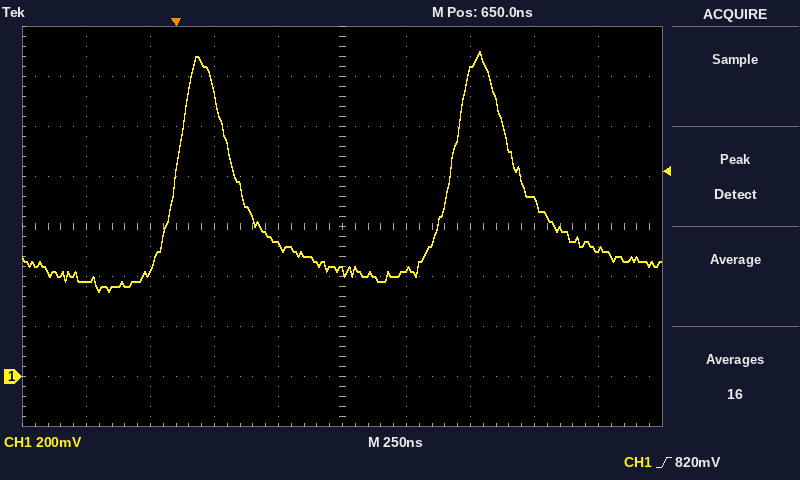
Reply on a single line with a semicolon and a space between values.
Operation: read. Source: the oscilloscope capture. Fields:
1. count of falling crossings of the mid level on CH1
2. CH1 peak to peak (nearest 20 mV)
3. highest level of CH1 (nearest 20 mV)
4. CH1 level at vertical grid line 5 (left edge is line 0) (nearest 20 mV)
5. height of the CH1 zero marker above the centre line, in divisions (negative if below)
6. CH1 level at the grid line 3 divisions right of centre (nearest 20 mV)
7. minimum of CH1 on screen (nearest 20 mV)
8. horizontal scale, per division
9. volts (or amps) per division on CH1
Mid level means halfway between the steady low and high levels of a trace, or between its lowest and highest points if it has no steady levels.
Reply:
2; 960 mV; 1.30 V; 420 mV; -3.0 div; 700 mV; 340 mV; 250 ns; 200 mV
